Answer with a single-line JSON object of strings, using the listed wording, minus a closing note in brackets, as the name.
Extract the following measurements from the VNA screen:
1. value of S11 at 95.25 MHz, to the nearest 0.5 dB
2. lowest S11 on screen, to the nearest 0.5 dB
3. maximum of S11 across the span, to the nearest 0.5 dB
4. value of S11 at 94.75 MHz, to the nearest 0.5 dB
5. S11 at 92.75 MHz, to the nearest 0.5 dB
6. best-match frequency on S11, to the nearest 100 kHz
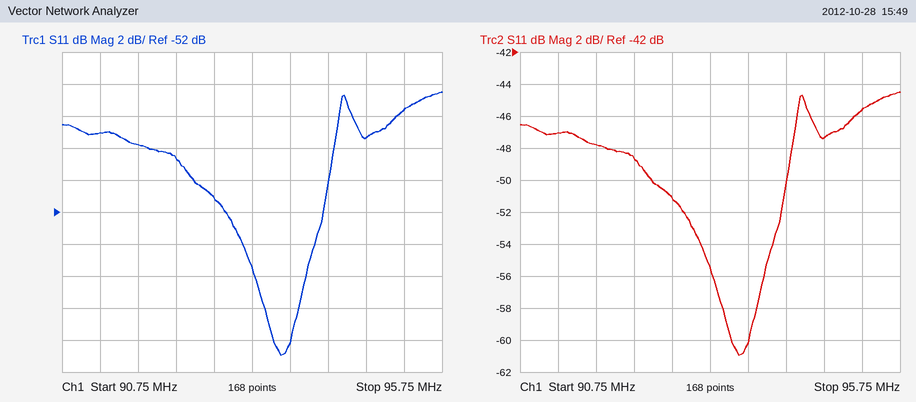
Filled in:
{"value of S11 at 95.25 MHz, to the nearest 0.5 dB": "-45.5 dB", "lowest S11 on screen, to the nearest 0.5 dB": "-61.0 dB", "maximum of S11 across the span, to the nearest 0.5 dB": "-44.5 dB", "value of S11 at 94.75 MHz, to the nearest 0.5 dB": "-47.5 dB", "S11 at 92.75 MHz, to the nearest 0.5 dB": "-51.0 dB", "best-match frequency on S11, to the nearest 100 kHz": "93.6 MHz"}
